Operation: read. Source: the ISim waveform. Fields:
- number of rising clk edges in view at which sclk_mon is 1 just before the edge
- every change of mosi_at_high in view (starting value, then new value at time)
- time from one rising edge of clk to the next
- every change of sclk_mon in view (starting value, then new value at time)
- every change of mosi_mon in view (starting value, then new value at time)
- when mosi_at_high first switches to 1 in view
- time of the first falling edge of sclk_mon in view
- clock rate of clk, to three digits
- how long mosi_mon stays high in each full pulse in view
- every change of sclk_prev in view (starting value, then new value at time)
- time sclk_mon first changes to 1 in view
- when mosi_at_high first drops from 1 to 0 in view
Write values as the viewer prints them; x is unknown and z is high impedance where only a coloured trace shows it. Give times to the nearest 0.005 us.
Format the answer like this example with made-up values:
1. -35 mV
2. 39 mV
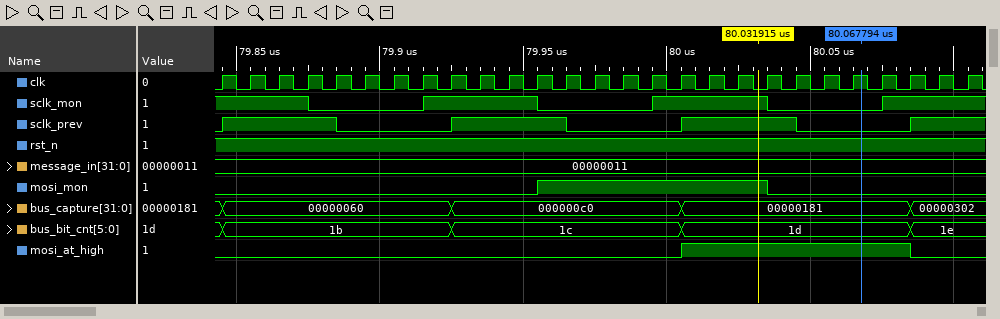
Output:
1. 15
2. 0, 1 at 80.005 us, 0 at 80.085 us
3. 0.01 us
4. 1, 0 at 79.875 us, 1 at 79.915 us, 0 at 79.955 us, 1 at 79.995 us, 0 at 80.035 us, 1 at 80.075 us
5. 0, 1 at 79.955 us, 0 at 80.035 us
6. 80.005 us
7. 79.875 us
8. 100 MHz
9. 0.08 us
10. 0, 1 at 79.845 us, 0 at 79.885 us, 1 at 79.925 us, 0 at 79.965 us, 1 at 80.005 us, 0 at 80.045 us, 1 at 80.085 us
11. 79.915 us
12. 80.085 us
